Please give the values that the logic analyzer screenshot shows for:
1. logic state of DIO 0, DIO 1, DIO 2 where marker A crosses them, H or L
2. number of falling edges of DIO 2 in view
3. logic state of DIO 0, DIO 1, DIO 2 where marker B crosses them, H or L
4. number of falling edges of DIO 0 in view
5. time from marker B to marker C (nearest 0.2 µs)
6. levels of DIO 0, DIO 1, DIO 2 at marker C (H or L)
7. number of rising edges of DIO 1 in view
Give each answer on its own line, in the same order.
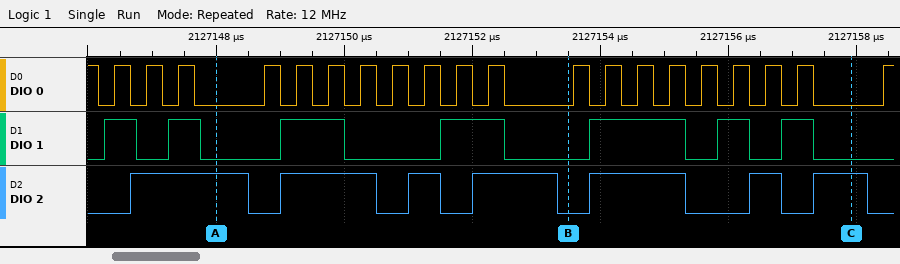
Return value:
DIO 0=L, DIO 1=L, DIO 2=H
7
DIO 0=L, DIO 1=L, DIO 2=L
20
4.4 µs
DIO 0=L, DIO 1=L, DIO 2=H
7
